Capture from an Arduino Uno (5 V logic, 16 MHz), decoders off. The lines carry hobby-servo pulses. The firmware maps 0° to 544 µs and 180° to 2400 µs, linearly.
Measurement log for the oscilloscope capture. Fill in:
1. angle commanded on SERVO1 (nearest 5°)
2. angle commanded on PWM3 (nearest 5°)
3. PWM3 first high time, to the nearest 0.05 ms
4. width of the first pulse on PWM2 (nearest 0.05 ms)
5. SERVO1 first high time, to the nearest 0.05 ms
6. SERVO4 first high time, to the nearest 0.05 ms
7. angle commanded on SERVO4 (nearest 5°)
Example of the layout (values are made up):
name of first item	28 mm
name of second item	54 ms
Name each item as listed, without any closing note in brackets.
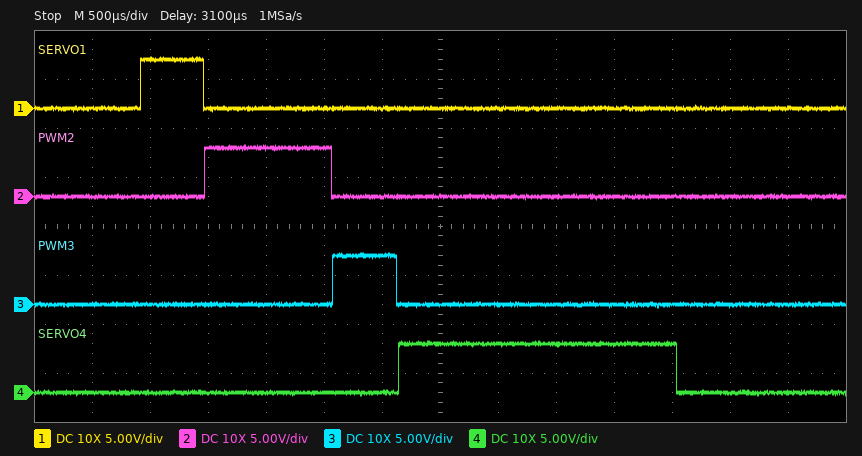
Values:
angle commanded on SERVO1	0°
angle commanded on PWM3	0°
PWM3 first high time, to the nearest 0.05 ms	0.55 ms
width of the first pulse on PWM2	1.10 ms
SERVO1 first high time, to the nearest 0.05 ms	0.55 ms
SERVO4 first high time, to the nearest 0.05 ms	2.40 ms
angle commanded on SERVO4	180°
